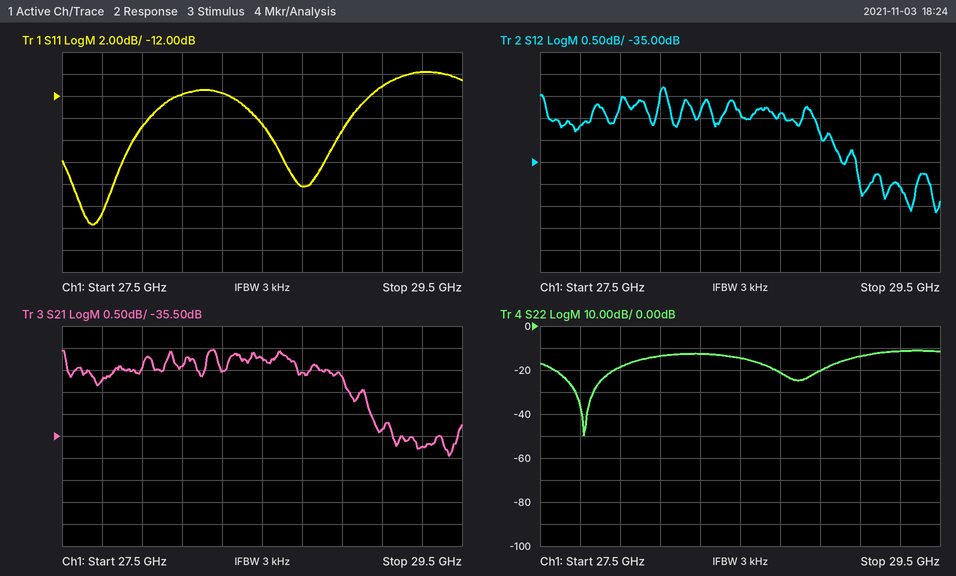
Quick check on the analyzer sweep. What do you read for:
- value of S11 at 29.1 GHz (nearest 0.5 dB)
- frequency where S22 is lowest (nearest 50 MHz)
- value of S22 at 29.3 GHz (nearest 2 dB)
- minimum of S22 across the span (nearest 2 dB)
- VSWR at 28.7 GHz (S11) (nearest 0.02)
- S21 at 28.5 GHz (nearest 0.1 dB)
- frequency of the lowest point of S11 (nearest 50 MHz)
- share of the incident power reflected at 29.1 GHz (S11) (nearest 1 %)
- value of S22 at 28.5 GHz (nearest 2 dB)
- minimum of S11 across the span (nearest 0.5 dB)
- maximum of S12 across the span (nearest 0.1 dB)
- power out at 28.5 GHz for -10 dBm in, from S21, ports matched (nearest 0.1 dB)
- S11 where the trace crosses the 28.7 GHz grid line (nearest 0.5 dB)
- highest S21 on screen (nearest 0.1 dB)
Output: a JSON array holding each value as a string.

["-11.0 dB", "27.70 GHz", "-12 dB", "-50 dB", "1.22", "-33.7 dB", "27.65 GHz", "8 %", "-14 dB", "-23.5 dB", "-33.3 dB", "-43.7 dBm", "-20.0 dB", "-33.5 dB"]
